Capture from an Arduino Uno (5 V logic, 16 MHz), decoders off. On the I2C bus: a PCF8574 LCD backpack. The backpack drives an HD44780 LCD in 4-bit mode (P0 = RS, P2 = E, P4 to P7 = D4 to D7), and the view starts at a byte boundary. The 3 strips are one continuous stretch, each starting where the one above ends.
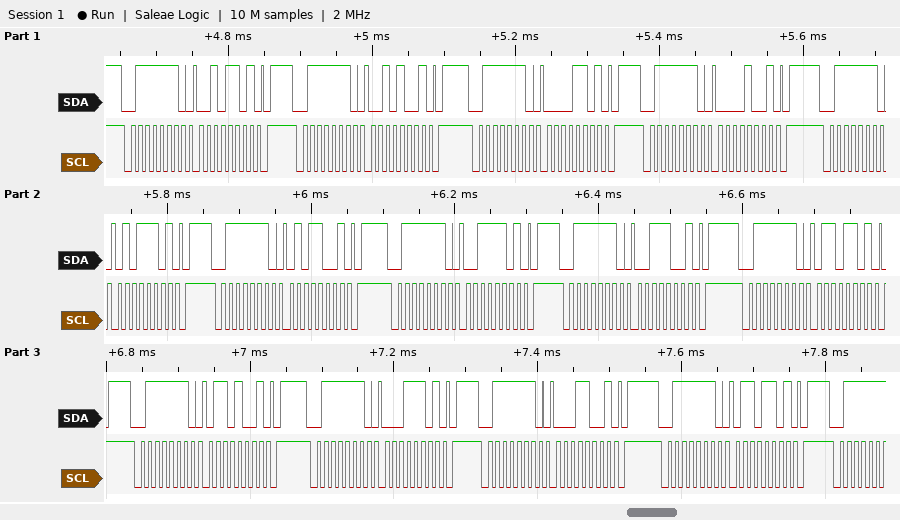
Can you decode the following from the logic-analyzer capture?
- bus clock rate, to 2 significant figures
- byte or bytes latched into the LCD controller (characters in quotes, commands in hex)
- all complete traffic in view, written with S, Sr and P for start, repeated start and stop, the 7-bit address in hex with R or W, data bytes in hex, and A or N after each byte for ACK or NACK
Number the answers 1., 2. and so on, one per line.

1. 100 kHz
2. ' ' 'S' 'a'
3. S 3FW A 2D A P S 3FW A 29 A P S 3FW A 0D A P S 3FW A 09 A P S 3FW A 5D A P S 3FW A 59 A P S 3FW A 3D A P S 3FW A 39 A P S 3FW A 6D A P S 3FW A 69 A P S 3FW A 1D A P S 3FW A 19 A P S 3FW A 6D A P
